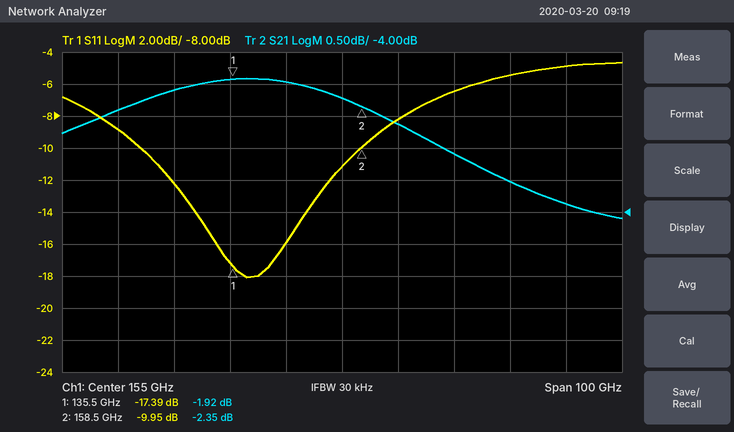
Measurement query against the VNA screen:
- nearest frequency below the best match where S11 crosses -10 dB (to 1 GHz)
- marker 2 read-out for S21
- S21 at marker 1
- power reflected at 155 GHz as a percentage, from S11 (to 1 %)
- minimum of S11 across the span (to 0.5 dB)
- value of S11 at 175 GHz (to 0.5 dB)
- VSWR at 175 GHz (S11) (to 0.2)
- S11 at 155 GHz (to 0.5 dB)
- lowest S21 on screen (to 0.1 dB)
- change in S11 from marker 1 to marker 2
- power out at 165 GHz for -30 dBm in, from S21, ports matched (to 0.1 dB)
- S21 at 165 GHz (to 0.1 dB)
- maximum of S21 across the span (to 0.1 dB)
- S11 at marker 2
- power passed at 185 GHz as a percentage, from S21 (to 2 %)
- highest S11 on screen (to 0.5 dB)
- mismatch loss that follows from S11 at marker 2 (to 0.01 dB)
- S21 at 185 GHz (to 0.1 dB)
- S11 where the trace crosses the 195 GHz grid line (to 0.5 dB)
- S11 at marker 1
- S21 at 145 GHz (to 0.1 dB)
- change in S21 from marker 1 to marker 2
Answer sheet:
119 GHz
-2.35 dB
-1.92 dB
8 %
-18.0 dB
-6.5 dB
2.8
-11.0 dB
-4.1 dB
7.44 dB
-32.6 dBm
-2.6 dB
-1.9 dB
-9.95 dB
44 %
-4.5 dB
0.46 dB
-3.5 dB
-5.0 dB
-17.39 dB
-2.0 dB
-0.43 dB
